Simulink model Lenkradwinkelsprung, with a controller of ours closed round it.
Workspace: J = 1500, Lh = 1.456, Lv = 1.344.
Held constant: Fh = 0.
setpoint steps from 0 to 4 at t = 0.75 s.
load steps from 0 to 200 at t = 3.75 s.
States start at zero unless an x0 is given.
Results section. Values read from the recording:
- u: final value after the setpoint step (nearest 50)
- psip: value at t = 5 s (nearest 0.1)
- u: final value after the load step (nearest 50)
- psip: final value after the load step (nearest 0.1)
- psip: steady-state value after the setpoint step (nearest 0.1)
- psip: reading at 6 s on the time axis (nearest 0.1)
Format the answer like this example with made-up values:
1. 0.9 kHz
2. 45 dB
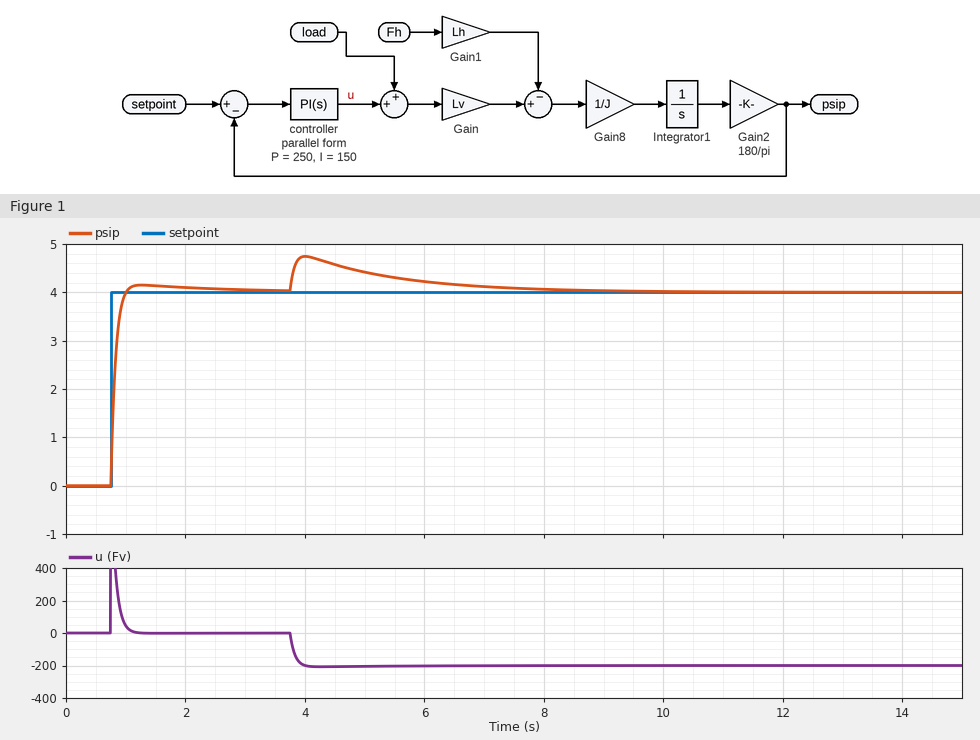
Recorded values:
1. 0
2. 4.4
3. -200
4. 4.0
5. 4.0
6. 4.2
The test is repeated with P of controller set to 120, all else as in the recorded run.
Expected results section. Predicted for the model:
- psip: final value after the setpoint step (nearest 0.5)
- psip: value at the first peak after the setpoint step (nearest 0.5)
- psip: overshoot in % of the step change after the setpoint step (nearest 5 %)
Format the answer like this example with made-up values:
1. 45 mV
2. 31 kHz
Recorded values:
1. 4.0
2. 4.5
3. 10 %
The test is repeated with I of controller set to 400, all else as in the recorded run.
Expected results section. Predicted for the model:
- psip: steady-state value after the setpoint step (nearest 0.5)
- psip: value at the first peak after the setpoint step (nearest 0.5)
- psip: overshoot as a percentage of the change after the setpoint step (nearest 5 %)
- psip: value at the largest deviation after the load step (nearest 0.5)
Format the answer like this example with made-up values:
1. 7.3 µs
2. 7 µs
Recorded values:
1. 4.0
2. 4.5
3. 10 %
4. 4.5
